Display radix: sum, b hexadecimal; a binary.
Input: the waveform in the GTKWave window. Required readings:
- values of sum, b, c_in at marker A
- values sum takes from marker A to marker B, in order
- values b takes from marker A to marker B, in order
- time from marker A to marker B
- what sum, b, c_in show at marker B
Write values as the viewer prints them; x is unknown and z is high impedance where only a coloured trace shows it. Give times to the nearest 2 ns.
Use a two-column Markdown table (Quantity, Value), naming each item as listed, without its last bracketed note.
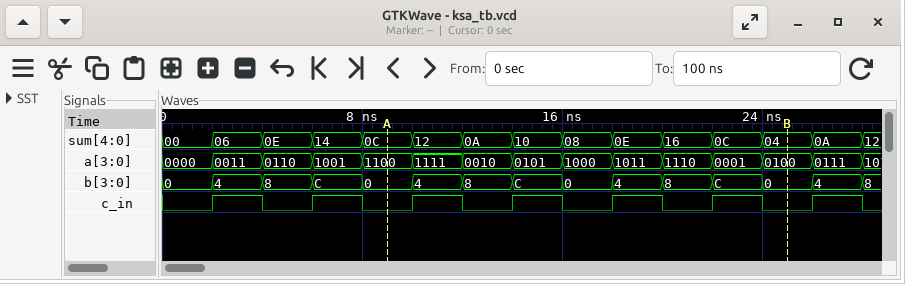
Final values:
| Quantity | Value |
|---|---|
| values of sum, b, c_in at marker A | sum=0C, b=0, c_in=0 |
| values sum takes from marker A to marker B, in order | 0C, 12, 0A, 10, 08, 0E, 16, 0C, 04 |
| values b takes from marker A to marker B, in order | 0, 4, 8, C, 0, 4, 8, C, 0 |
| time from marker A to marker B | 16 ns |
| what sum, b, c_in show at marker B | sum=04, b=0, c_in=0 |
